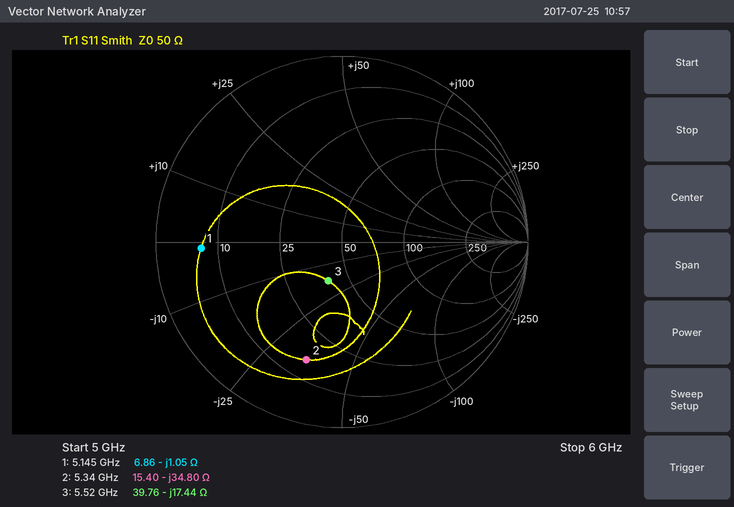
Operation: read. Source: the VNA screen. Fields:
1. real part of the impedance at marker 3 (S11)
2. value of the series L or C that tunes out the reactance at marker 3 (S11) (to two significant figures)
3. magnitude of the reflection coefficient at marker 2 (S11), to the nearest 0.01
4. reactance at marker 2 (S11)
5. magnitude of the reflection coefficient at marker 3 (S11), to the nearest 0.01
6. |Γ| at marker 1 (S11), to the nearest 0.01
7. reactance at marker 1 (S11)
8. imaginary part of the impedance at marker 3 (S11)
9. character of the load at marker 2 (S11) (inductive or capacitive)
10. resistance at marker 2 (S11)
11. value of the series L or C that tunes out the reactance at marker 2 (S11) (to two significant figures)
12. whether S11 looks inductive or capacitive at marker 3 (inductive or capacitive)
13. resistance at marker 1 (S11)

39.76 Ω
500 pH
0.66
-34.80 Ω
0.22
0.76
-1.05 Ω
-17.44 Ω
capacitive
15.40 Ω
1.0 nH
capacitive
6.86 Ω
